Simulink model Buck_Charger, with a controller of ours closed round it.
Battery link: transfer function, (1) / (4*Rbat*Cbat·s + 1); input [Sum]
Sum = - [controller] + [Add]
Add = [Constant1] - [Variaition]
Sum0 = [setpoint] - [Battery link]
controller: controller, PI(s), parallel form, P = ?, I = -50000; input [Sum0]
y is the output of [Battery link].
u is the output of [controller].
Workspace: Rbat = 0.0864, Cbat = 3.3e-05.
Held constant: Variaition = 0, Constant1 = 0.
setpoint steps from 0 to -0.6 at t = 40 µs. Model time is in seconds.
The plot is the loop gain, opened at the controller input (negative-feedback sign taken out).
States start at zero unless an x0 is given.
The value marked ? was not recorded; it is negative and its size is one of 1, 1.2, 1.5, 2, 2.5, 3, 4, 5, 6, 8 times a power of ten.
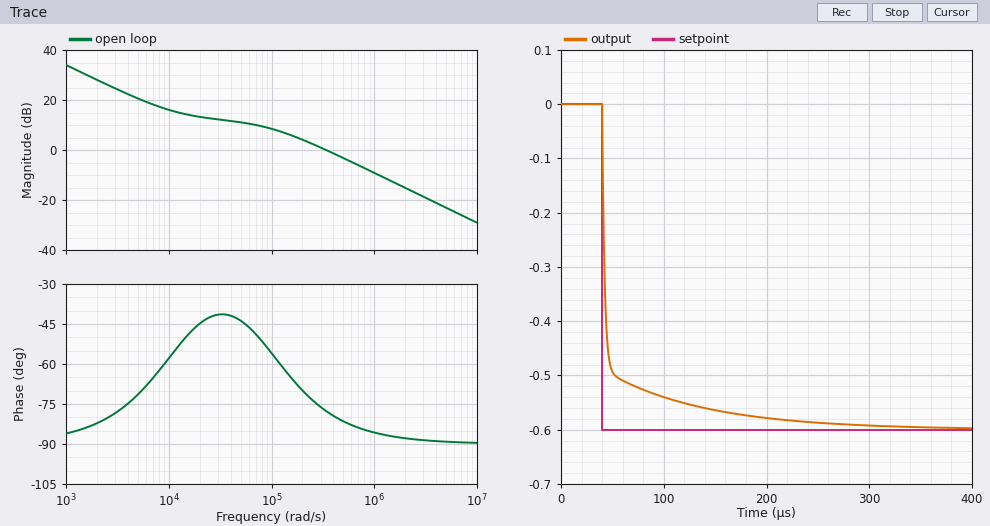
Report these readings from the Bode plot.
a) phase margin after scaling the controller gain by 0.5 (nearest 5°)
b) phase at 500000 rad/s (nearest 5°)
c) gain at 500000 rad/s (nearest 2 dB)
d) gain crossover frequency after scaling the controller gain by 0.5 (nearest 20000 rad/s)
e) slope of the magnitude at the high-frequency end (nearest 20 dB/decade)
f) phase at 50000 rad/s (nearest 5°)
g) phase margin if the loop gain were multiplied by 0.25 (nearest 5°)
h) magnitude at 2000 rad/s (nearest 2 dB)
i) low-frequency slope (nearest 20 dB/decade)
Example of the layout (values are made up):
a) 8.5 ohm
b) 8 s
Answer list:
a) 115°
b) -80°
c) -4 dB
d) 160000 rad/s
e) -20 dB/decade
f) -45°
g) 140°
h) 28 dB
i) -20 dB/decade
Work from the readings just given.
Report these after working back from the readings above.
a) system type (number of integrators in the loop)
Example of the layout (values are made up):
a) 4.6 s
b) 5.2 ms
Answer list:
a) 1
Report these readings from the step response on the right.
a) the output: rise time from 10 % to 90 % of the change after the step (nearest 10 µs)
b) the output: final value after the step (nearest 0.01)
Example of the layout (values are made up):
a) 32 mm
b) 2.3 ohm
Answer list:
a) 60 µs
b) -0.60
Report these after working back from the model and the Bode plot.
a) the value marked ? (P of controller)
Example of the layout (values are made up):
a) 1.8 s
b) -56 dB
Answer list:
a) -4
